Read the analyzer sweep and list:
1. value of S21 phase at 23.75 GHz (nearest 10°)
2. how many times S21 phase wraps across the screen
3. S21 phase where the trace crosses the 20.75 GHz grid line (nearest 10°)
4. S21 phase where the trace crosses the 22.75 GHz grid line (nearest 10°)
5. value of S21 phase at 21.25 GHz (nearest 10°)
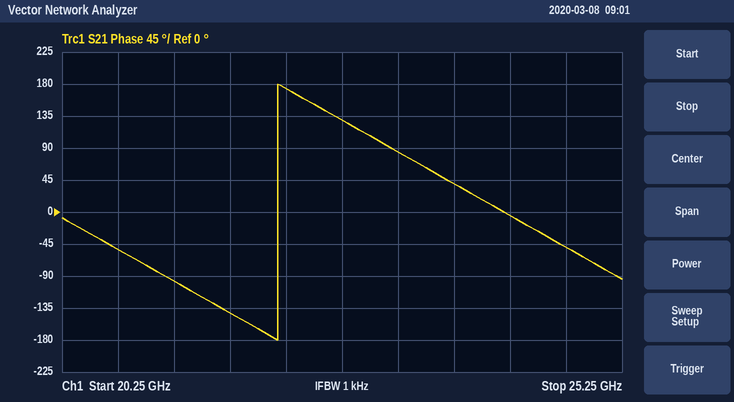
40°
1
-50°
130°
-100°
